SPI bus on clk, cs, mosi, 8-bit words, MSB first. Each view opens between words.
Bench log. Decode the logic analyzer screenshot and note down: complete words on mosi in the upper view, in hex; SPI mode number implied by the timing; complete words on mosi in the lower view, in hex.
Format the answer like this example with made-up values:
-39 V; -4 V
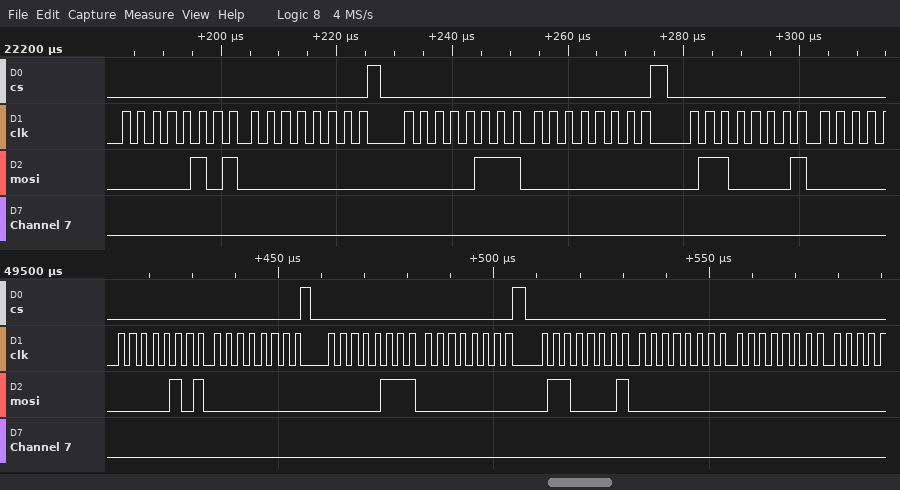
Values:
05, 00, 07, 00, 61; 0; 05, 00, 07, 00, 61, 00, 00
